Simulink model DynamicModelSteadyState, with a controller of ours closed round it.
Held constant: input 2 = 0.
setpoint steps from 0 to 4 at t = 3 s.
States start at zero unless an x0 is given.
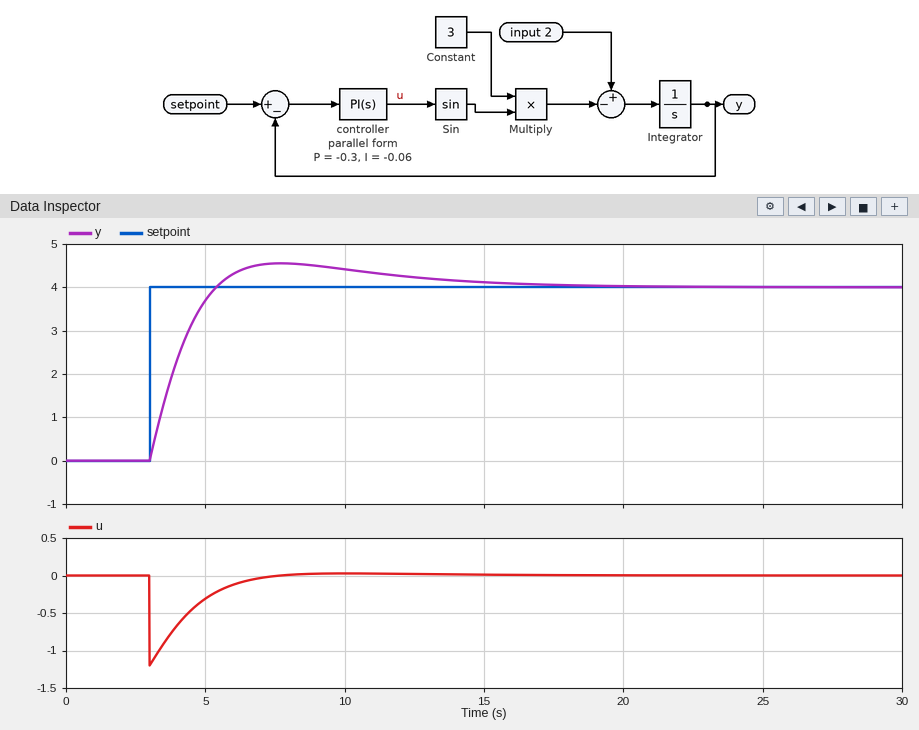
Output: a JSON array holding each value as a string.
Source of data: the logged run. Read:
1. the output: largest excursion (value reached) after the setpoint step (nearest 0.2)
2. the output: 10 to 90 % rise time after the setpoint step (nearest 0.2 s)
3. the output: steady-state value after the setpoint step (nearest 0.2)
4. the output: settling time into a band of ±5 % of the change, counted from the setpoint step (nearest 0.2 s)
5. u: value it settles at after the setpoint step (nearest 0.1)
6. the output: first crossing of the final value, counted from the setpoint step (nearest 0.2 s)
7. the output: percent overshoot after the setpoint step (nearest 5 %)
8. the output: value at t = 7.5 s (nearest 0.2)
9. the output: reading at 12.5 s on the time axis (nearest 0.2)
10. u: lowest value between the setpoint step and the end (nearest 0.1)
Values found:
["4.6", "1.8 s", "4.0", "10.0 s", "0.0", "2.4 s", "15 %", "4.6", "4.2", "-1.2"]
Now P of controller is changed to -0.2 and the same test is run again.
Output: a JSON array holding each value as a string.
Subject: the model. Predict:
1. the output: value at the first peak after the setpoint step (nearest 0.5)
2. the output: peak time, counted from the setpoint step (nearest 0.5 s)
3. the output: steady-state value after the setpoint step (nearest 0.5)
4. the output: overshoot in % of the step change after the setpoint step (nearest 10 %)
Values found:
["5.0", "5.5 s", "4.0", "20 %"]
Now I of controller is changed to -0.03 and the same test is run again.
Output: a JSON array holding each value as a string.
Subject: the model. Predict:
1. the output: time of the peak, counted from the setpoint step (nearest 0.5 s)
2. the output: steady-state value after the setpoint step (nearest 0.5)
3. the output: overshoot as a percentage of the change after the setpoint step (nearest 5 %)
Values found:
["6.0 s", "4.0", "10 %"]
